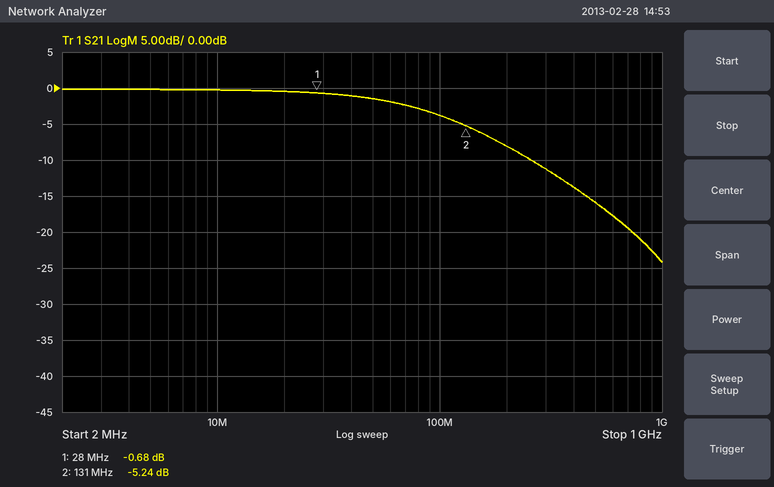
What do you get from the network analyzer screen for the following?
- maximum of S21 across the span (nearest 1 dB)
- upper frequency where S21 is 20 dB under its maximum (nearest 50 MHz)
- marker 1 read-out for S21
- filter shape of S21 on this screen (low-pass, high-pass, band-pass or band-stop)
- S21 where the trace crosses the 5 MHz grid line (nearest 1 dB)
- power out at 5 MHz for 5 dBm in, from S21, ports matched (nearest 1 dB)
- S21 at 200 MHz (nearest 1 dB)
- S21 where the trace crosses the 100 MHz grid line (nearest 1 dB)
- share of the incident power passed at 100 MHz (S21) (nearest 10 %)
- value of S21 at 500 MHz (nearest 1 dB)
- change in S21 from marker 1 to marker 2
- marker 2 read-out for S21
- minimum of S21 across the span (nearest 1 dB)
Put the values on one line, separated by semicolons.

0 dB; 750 MHz; -0.68 dB; low-pass; 0 dB; 5 dBm; -8 dB; -4 dB; 40 %; -16 dB; -4.56 dB; -5.24 dB; -24 dB
